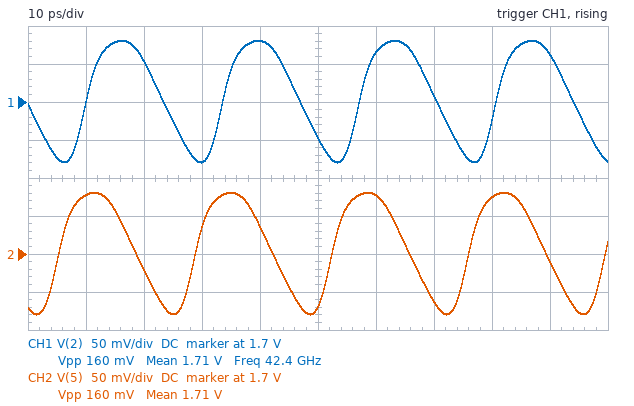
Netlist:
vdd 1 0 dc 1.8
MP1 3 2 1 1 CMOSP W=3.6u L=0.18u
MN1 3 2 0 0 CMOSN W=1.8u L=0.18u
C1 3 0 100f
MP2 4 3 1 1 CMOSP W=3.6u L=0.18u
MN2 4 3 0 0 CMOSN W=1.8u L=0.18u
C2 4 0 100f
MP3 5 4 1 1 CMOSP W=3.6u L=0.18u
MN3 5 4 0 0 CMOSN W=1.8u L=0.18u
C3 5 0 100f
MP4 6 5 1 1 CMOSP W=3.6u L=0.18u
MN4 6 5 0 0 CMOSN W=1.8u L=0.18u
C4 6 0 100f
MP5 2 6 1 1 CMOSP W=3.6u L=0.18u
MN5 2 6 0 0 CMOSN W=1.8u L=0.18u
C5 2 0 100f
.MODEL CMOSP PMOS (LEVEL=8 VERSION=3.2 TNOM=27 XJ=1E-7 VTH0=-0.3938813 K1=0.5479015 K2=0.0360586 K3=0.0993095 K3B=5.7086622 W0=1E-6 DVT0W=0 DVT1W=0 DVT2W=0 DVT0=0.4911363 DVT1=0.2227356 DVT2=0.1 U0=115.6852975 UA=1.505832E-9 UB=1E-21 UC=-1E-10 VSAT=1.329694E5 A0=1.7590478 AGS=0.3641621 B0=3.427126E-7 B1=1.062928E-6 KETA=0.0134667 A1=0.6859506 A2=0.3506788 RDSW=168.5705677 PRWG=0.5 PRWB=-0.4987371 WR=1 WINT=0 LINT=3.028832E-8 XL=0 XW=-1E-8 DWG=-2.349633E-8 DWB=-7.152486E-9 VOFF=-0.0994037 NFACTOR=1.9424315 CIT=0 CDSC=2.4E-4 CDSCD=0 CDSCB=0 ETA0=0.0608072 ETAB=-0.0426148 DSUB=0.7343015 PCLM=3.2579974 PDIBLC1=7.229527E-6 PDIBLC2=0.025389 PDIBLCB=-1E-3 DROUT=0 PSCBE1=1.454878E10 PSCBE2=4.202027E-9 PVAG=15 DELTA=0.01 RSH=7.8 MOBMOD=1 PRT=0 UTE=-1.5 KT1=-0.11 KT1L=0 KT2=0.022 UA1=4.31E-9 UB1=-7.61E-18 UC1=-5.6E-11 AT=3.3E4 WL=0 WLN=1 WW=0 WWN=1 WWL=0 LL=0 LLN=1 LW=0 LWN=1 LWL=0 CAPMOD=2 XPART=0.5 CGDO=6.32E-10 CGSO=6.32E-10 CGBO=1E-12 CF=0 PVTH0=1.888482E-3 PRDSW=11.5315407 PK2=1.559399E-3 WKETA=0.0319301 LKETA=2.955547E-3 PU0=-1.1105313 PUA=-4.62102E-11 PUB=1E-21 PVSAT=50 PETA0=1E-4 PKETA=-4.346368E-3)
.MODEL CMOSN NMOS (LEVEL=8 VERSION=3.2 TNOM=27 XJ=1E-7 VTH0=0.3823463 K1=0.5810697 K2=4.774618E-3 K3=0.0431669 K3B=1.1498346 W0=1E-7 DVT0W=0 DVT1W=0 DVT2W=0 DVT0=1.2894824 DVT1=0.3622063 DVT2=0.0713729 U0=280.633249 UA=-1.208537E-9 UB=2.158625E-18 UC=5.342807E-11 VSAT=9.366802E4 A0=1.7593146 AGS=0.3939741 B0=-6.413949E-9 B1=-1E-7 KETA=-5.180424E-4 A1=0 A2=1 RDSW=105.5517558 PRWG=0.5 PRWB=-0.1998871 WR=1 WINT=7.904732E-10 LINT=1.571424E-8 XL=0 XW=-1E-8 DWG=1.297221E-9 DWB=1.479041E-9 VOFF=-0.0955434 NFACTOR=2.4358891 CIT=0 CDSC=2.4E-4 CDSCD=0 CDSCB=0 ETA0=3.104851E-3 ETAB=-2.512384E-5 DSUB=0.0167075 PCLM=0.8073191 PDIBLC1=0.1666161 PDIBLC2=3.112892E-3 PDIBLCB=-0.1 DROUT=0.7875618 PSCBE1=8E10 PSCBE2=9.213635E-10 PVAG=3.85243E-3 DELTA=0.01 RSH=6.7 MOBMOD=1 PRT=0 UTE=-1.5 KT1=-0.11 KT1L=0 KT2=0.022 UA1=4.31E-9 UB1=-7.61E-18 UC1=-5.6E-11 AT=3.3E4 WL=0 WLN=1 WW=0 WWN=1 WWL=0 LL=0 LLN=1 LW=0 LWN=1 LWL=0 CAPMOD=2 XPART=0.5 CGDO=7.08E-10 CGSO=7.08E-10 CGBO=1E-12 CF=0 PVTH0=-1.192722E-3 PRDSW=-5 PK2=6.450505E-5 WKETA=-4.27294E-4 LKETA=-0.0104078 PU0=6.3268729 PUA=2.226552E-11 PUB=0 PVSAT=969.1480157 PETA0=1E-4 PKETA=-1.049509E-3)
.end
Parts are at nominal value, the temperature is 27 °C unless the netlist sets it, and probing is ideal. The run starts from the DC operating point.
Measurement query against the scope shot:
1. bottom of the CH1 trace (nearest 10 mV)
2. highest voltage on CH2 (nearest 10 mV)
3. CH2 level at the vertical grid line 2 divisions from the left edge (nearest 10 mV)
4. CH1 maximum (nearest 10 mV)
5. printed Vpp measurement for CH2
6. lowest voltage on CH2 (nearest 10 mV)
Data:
1.62 V
1.78 V
1.68 V
1.78 V
160 mV
1.62 V
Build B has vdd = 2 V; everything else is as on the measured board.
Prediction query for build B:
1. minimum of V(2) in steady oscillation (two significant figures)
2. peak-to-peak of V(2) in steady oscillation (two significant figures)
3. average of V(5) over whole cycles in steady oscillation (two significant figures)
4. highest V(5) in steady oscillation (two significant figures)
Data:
1.8 V
180 mV
1.9 V
2.0 V
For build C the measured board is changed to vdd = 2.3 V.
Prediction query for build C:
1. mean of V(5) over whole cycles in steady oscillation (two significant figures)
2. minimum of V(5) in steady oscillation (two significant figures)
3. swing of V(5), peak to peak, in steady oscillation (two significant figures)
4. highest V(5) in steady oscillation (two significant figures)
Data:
2.2 V
2.1 V
200 mV
2.3 V
